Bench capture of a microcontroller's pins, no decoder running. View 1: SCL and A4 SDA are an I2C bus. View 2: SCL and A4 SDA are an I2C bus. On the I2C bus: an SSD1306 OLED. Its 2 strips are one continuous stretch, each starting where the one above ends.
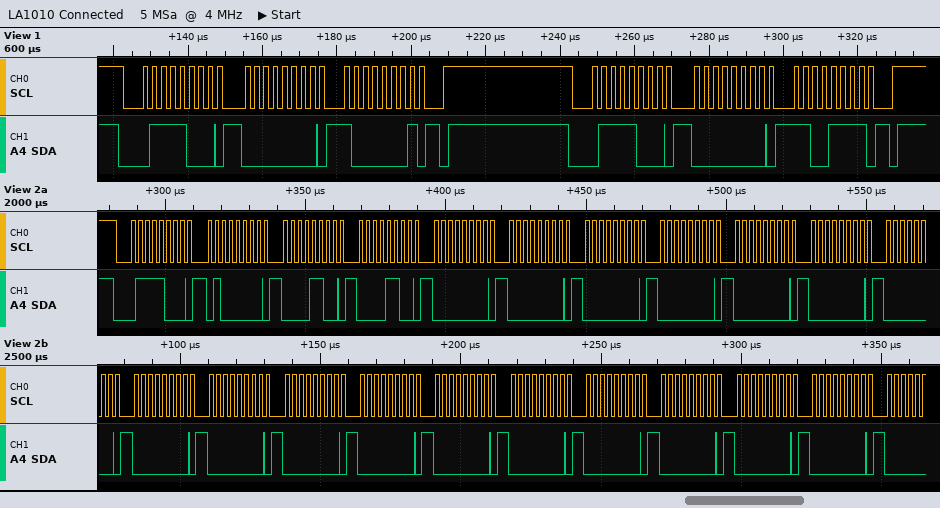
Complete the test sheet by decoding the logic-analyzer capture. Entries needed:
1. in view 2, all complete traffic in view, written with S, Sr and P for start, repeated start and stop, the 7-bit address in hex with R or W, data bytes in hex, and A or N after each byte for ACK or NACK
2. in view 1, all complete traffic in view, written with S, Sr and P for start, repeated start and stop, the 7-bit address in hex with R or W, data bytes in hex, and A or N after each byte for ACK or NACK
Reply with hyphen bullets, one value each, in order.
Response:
- S 3CW A 40 A 0C A 0C A 00 A 00 A 00 A 00 A 00 A 00 A 00 A 00 A 00 A 00 A 00 A 00 A 00 A 00 A 00 A 00 A 00 A
- S 3CW A 00 A 81 A P S 3CW A 00 A CF A P
